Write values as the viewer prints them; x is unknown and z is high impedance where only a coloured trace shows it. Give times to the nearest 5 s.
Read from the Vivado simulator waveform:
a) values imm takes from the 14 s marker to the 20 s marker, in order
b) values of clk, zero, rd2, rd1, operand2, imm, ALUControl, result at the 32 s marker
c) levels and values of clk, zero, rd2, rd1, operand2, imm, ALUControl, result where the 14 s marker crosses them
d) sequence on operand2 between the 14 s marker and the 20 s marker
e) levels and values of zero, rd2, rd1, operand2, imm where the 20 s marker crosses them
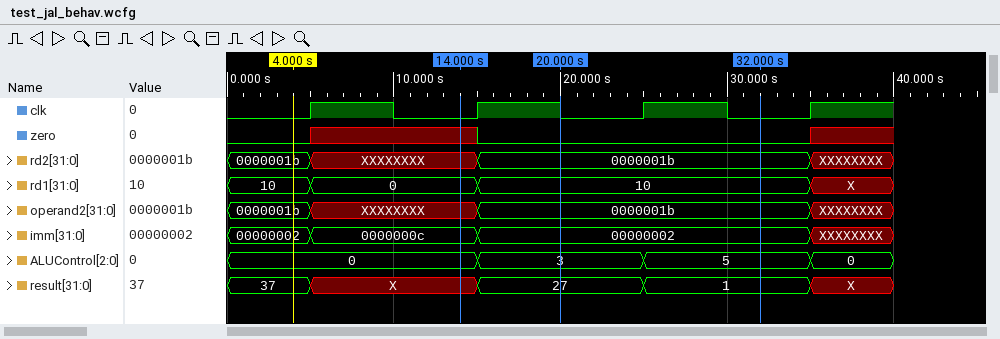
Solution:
0000000c, 00000002
clk=0, zero=0, rd2=0000001b, rd1=10, operand2=0000001b, imm=00000002, ALUControl=5, result=1
clk=0, zero=x, rd2=XXXXXXXX, rd1=0, operand2=XXXXXXXX, imm=0000000c, ALUControl=0, result=X
XXXXXXXX, 0000001b
zero=0, rd2=0000001b, rd1=10, operand2=0000001b, imm=00000002
